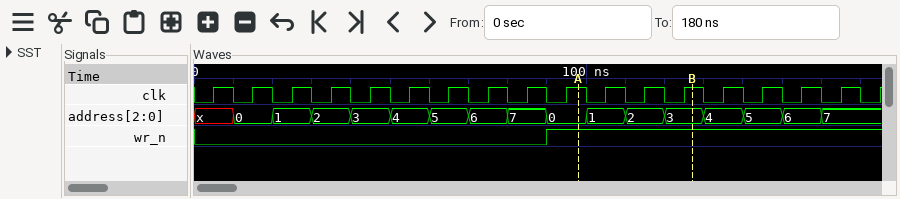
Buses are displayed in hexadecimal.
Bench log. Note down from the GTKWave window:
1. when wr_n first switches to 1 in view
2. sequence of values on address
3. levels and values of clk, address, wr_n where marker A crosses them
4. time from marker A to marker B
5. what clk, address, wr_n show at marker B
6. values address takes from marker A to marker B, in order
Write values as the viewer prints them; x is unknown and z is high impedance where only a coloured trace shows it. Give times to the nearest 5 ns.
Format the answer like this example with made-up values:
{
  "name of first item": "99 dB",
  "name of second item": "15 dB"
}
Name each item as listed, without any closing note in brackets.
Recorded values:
{
  "when wr_n first switches to 1 in view": "90 ns",
  "sequence of values on address": "x, 0, 1, 2, 3, 4, 5, 6, 7, 0, 1, 2, 3, 4, 5, 6, 7",
  "levels and values of clk, address, wr_n where marker A crosses them": "clk=1, address=0, wr_n=1",
  "time from marker A to marker B": "30 ns",
  "what clk, address, wr_n show at marker B": "clk=1, address=3, wr_n=1",
  "values address takes from marker A to marker B, in order": "0, 1, 2, 3"
}
